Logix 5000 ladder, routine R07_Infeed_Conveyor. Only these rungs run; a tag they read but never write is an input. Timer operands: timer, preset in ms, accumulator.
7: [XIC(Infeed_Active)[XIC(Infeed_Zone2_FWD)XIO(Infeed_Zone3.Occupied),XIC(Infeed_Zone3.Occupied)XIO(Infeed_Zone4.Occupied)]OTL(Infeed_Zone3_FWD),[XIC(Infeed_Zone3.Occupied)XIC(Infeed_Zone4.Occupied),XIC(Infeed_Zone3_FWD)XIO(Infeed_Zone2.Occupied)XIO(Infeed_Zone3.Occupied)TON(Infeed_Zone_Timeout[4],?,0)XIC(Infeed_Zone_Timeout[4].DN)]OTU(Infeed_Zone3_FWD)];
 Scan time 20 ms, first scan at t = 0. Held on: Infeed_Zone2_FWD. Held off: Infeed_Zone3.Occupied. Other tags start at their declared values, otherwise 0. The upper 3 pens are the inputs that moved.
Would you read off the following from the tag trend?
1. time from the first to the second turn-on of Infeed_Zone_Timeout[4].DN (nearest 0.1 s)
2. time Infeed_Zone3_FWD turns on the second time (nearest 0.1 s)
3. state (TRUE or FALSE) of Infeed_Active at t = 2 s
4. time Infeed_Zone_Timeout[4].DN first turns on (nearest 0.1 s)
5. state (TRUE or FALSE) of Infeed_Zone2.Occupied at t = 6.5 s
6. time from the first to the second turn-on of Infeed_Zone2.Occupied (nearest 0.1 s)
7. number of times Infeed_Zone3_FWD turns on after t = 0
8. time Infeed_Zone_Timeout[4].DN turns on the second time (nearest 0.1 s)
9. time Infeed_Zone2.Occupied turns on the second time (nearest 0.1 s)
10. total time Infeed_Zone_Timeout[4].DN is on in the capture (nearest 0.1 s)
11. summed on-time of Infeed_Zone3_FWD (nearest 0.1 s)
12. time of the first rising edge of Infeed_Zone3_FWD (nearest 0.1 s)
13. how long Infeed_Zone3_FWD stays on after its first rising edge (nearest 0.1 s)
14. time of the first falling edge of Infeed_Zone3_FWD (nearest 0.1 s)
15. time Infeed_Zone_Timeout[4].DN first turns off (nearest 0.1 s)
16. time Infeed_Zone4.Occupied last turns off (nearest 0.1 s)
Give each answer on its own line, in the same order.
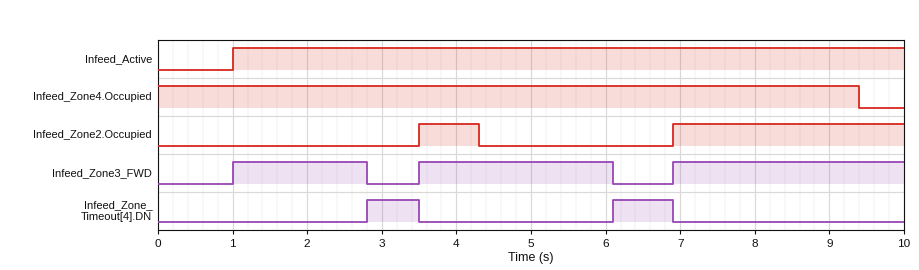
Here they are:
3.3 s
3.5 s
TRUE
2.8 s
FALSE
3.4 s
3
6.1 s
6.9 s
1.5 s
7.5 s
1.0 s
1.8 s
2.8 s
3.5 s
9.4 s
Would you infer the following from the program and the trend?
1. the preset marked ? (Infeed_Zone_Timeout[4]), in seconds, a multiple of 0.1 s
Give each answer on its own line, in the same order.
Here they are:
1.8 s
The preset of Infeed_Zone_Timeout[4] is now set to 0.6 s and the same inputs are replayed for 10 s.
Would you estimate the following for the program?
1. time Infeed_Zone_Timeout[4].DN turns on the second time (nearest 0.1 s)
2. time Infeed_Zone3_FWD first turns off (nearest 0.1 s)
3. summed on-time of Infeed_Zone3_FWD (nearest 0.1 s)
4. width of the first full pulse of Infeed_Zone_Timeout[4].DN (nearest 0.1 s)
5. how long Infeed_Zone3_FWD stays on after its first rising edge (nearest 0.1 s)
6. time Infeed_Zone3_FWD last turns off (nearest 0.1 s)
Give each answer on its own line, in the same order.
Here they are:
4.9 s
1.6 s
5.1 s
1.9 s
0.6 s
4.9 s
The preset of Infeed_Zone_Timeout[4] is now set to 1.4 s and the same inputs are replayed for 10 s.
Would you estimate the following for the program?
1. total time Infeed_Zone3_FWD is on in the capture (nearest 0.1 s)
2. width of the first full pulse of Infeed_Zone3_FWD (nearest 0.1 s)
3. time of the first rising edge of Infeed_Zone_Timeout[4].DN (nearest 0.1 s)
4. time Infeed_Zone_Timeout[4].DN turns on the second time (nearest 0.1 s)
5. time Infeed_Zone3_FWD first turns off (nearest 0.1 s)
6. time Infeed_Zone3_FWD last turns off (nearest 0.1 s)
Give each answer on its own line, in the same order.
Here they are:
6.7 s
1.4 s
2.4 s
5.7 s
2.4 s
5.7 s
